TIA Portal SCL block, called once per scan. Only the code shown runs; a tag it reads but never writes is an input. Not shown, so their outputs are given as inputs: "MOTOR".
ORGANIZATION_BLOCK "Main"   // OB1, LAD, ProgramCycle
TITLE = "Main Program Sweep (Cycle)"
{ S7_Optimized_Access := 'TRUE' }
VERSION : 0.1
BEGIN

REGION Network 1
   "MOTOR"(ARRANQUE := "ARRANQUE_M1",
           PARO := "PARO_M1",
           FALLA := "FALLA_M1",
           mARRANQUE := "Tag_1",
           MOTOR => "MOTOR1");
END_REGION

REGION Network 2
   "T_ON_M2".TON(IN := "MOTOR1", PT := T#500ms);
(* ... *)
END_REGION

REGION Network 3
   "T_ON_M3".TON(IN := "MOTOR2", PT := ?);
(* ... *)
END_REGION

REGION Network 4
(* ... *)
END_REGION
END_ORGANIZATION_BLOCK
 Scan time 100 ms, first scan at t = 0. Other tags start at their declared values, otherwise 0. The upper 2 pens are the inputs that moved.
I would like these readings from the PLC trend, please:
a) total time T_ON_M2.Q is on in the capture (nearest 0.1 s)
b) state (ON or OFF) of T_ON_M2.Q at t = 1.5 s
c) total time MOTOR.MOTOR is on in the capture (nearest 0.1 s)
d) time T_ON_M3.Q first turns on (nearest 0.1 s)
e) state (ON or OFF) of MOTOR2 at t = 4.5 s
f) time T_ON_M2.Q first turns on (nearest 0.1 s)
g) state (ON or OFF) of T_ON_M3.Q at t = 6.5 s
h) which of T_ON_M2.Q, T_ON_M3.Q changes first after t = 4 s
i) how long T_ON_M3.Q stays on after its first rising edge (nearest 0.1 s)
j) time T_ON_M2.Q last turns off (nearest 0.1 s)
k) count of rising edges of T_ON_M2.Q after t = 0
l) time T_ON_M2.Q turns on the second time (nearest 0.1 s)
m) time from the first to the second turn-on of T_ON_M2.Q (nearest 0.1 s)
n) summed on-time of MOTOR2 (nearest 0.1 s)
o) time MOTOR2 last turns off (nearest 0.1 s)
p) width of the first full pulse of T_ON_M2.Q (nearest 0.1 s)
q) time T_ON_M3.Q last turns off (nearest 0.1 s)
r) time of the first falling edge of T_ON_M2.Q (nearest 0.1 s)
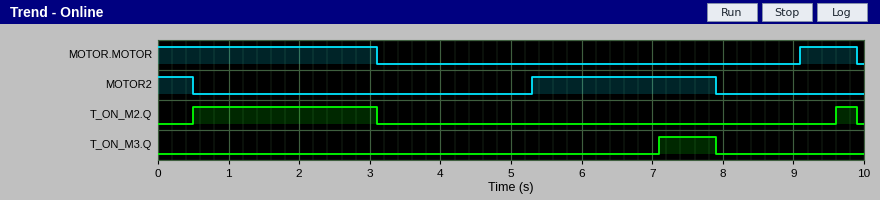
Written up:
2.9 s
ON
3.9 s
7.1 s
OFF
0.5 s
OFF
T_ON_M3.Q
0.8 s
9.9 s
2
9.6 s
9.1 s
3.1 s
7.9 s
2.6 s
7.9 s
3.1 s
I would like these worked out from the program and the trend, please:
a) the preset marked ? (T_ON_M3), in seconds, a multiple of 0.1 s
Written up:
1.8 s
